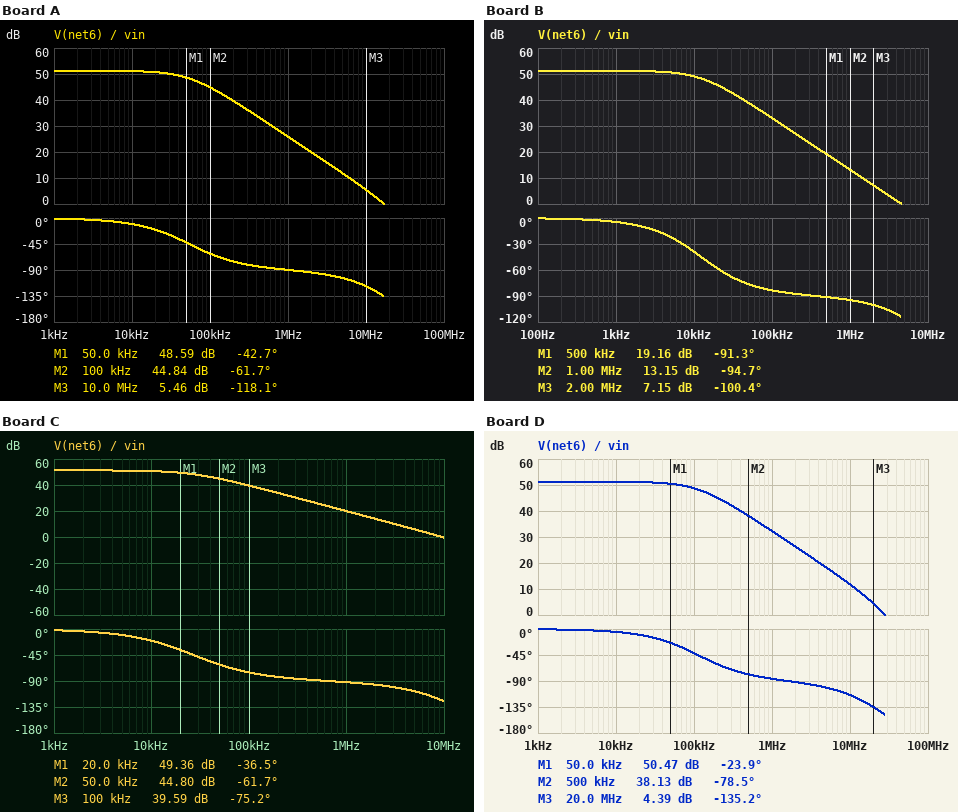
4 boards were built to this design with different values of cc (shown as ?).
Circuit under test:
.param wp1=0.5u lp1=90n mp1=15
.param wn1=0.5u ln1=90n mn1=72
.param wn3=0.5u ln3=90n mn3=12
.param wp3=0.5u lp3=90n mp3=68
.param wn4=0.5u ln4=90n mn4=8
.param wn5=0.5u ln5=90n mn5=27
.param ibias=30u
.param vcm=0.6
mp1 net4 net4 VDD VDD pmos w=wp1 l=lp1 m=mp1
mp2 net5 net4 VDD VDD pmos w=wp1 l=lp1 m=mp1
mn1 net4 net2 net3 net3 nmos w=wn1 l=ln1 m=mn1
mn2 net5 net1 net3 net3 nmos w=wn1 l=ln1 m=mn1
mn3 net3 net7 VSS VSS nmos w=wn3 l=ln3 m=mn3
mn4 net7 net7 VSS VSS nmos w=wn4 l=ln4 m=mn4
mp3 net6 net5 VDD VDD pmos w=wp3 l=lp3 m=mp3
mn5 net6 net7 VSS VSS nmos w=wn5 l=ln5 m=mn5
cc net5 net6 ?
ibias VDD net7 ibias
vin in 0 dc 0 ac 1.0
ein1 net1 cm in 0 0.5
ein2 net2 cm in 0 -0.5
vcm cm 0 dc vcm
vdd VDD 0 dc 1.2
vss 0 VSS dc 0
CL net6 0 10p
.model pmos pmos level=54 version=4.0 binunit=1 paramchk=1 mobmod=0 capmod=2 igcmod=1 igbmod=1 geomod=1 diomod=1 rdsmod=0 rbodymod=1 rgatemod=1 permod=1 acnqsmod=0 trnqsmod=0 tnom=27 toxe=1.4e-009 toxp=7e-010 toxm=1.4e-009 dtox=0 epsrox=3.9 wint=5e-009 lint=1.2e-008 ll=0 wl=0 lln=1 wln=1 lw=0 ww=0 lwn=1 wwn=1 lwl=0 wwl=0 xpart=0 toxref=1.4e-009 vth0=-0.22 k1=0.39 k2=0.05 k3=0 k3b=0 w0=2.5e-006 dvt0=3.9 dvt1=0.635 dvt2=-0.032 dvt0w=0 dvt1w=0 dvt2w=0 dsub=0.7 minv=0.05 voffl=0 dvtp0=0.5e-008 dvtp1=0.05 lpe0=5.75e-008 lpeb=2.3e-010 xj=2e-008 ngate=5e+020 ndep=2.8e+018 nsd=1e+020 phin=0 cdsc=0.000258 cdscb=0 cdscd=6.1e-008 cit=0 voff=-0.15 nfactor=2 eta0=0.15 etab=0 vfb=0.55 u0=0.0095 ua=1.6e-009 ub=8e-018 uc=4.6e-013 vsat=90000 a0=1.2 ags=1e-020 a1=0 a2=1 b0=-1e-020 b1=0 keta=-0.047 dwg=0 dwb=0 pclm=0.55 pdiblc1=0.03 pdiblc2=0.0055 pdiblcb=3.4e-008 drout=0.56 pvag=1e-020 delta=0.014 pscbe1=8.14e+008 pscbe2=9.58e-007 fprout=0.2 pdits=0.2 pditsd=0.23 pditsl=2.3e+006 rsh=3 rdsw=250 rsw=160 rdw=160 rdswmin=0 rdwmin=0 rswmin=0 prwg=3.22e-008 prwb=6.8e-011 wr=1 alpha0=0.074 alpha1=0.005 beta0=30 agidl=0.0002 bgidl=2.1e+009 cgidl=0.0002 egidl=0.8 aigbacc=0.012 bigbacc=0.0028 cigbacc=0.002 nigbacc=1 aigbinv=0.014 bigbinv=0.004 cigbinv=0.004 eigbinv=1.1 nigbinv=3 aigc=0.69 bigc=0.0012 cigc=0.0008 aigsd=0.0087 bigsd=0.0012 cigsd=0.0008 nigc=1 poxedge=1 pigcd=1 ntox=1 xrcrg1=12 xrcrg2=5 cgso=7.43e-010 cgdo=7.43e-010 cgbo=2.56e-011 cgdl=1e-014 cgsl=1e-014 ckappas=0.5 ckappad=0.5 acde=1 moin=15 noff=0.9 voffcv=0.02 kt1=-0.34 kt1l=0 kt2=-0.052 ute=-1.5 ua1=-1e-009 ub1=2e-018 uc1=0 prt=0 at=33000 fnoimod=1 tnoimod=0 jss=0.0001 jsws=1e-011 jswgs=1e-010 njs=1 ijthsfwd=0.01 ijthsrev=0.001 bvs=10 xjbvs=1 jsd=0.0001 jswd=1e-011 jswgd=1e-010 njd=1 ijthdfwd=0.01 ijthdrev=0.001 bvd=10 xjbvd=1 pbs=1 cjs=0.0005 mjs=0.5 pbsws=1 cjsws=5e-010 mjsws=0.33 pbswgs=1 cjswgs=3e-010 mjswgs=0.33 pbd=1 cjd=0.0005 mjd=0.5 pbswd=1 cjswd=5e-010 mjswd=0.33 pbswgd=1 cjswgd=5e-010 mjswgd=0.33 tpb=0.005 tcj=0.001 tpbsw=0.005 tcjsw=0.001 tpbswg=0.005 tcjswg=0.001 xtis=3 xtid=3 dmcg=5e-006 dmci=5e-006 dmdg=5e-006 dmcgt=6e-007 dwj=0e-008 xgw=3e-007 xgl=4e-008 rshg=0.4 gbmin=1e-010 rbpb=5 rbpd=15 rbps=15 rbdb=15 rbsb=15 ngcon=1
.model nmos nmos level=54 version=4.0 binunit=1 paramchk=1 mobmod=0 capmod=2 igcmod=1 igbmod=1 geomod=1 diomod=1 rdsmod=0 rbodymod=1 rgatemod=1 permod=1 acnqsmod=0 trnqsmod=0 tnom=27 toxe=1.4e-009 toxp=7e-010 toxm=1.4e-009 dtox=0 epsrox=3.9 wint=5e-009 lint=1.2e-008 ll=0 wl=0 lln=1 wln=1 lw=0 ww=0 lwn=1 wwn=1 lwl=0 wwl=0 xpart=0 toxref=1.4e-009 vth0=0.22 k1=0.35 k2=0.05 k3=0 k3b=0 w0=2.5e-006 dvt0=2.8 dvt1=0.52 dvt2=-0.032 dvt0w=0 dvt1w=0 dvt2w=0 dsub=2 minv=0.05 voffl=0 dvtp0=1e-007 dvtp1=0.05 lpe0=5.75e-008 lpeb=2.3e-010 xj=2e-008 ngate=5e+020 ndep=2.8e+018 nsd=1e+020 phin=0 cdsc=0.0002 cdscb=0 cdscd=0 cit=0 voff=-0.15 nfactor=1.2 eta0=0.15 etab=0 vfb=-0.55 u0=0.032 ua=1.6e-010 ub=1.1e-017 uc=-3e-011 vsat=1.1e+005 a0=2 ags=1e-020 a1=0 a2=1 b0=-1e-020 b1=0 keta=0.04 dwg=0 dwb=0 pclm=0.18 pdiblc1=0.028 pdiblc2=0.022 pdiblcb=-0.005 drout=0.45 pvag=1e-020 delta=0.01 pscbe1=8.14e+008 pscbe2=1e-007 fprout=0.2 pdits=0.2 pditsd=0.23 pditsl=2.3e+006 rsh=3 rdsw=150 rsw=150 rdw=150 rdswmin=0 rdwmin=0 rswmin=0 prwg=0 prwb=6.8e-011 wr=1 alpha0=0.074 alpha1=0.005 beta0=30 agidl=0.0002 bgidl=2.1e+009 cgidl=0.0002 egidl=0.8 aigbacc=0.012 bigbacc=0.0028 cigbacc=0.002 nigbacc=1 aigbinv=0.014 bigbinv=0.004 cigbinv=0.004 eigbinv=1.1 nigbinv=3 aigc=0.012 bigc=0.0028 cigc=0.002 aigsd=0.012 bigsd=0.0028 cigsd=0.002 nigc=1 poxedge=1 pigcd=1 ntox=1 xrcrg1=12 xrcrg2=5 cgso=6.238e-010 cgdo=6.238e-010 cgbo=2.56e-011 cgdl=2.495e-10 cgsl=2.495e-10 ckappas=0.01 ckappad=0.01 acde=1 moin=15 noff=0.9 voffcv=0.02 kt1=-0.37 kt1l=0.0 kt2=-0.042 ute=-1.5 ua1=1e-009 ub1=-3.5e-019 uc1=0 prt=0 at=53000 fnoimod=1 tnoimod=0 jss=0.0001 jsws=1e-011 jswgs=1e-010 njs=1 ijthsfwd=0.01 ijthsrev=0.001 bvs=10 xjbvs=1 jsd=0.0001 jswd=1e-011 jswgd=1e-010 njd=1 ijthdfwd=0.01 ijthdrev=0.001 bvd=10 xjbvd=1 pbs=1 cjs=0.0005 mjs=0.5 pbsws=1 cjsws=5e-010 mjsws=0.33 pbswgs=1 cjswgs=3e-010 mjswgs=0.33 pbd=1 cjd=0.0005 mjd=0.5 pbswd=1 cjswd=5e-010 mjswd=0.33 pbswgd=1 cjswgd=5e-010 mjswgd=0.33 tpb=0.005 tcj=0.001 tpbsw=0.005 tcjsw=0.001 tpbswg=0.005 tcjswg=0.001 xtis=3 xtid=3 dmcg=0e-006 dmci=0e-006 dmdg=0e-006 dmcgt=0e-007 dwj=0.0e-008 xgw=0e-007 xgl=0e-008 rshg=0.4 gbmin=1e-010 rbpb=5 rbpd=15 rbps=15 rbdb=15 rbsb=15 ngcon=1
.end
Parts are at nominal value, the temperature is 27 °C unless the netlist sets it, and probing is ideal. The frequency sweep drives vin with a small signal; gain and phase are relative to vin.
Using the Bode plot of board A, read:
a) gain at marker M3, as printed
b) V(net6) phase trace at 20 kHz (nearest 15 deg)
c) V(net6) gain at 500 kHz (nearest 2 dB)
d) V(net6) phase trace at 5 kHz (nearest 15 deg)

5.46 dB
-15 deg
32 dB
0 deg
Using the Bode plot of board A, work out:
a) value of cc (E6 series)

3.3 pF
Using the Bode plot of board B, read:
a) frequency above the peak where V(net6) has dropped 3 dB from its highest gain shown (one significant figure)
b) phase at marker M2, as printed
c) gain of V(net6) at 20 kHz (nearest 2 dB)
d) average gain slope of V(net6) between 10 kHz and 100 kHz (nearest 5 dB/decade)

10 kHz
-94.7 deg
46 dB
-15 dB/decade
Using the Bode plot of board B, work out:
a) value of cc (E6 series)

15 pF
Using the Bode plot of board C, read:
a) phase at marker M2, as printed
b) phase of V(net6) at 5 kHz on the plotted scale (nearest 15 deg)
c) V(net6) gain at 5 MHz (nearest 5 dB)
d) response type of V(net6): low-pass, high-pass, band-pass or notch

-61.7 deg
-15 deg
5 dB
low-pass
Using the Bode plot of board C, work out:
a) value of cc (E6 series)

6.8 pF
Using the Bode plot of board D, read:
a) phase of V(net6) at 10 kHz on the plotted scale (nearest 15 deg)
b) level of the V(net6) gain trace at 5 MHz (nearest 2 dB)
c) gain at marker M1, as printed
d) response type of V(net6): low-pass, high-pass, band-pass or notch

0 deg
18 dB
50.47 dB
low-pass
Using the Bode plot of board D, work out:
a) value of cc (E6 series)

1.5 pF
